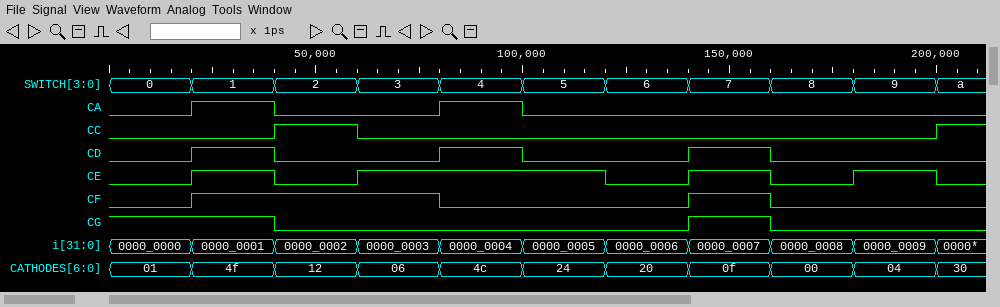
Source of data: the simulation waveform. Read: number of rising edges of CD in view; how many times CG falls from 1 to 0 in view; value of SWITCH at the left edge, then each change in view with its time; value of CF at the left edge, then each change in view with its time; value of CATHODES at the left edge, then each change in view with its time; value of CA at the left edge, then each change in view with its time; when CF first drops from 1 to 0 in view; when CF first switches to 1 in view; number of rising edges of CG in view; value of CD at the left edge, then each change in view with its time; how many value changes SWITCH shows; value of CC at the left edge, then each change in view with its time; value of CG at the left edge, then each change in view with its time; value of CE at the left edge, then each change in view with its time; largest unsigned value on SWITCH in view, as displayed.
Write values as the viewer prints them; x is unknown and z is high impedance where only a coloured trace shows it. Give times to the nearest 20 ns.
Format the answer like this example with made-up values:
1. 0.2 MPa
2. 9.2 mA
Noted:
1. 3
2. 2
3. 0, 1 at 20 ns, 2 at 40 ns, 3 at 60 ns, 4 at 80 ns, 5 at 100 ns, 6 at 120 ns, 7 at 140 ns, 8 at 160 ns, 9 at 180 ns, a at 200 ns
4. 0, 1 at 20 ns, 0 at 80 ns, 1 at 140 ns, 0 at 160 ns
5. 01, 4f at 20 ns, 12 at 40 ns, 06 at 60 ns, 4c at 80 ns, 24 at 100 ns, 20 at 120 ns, 0f at 140 ns, 00 at 160 ns, 04 at 180 ns, 30 at 200 ns
6. 0, 1 at 20 ns, 0 at 40 ns, 1 at 80 ns, 0 at 100 ns
7. 80 ns
8. 20 ns
9. 1
10. 0, 1 at 20 ns, 0 at 40 ns, 1 at 80 ns, 0 at 100 ns, 1 at 140 ns, 0 at 160 ns
11. 10
12. 0, 1 at 40 ns, 0 at 60 ns, 1 at 200 ns
13. 1, 0 at 40 ns, 1 at 140 ns, 0 at 160 ns
14. 0, 1 at 20 ns, 0 at 40 ns, 1 at 60 ns, 0 at 120 ns, 1 at 140 ns, 0 at 160 ns, 1 at 180 ns, 0 at 200 ns
15. a
